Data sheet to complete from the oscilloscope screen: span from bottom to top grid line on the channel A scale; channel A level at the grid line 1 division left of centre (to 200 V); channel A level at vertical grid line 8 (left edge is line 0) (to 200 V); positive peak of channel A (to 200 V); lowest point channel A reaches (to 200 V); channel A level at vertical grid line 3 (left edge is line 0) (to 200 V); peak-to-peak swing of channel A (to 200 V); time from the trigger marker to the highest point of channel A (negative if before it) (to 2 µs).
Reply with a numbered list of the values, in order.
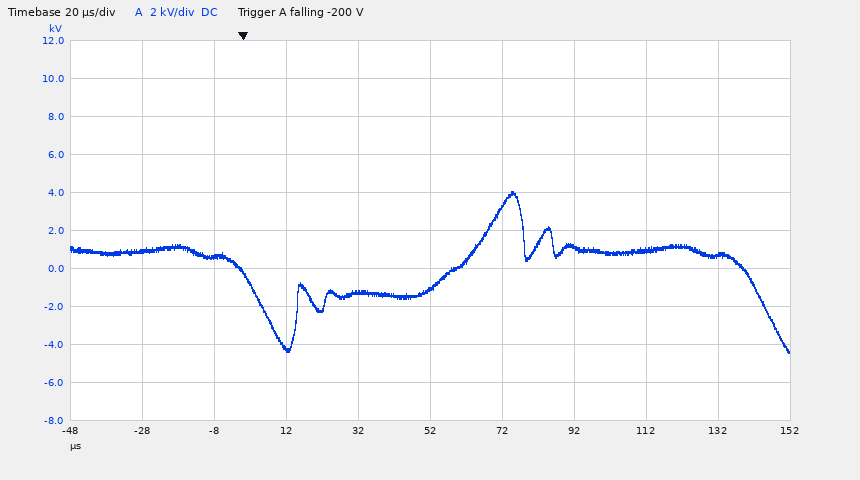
1. 20 kV
2. -1.2 kV
3. 1.0 kV
4. 4.0 kV
5. -4.4 kV
6. -4.2 kV
7. 8.4 kV
8. +74 µs
